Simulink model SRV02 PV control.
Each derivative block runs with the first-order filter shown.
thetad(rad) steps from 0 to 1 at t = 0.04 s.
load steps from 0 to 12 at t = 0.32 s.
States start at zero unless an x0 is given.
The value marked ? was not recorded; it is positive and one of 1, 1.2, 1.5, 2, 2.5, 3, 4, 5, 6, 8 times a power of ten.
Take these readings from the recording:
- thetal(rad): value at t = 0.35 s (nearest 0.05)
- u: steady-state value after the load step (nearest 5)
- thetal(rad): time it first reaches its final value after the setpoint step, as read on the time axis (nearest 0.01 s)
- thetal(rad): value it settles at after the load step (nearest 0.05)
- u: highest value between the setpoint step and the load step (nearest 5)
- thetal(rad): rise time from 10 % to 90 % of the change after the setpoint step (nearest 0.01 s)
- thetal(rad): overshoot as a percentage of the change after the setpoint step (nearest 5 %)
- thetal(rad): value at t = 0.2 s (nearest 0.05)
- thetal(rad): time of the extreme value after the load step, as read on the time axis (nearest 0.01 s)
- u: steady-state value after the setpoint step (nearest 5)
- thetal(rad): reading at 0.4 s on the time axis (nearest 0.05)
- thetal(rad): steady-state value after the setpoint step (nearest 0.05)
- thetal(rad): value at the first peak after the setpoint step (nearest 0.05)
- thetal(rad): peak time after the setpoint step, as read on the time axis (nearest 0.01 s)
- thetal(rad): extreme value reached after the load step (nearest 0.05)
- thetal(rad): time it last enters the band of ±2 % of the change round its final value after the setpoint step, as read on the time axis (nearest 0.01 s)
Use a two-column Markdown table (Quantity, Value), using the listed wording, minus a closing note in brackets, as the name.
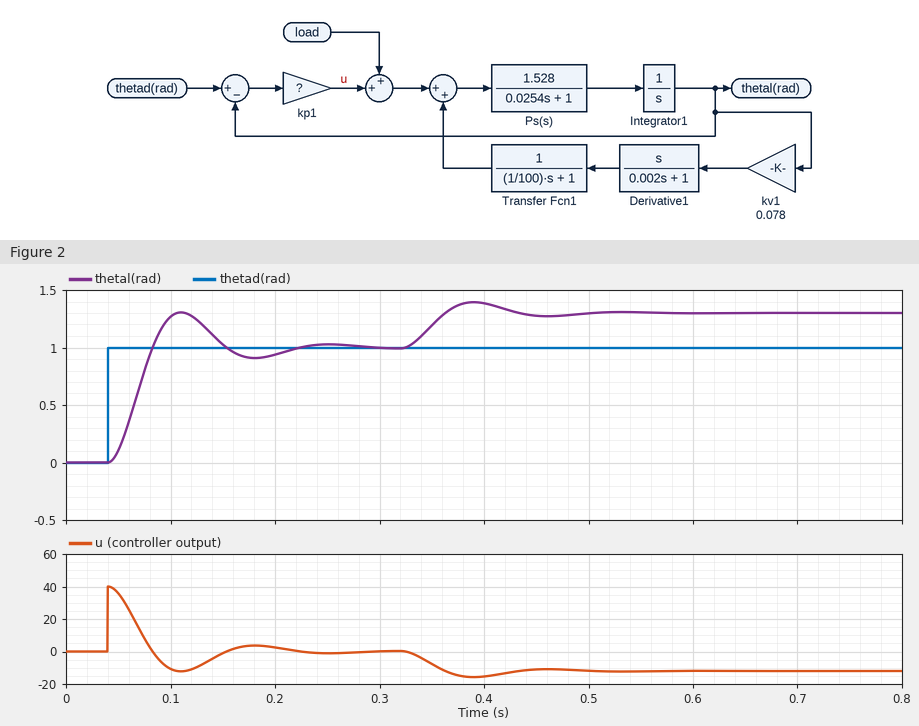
| Quantity | Value |
|---|---|
| thetal(rad): value at t = 0.35 s | 1.20 |
| u: steady-state value after the load step | -10 |
| thetal(rad): time it first reaches its final value after the setpoint step, as read on the time axis | 0.08 s |
| thetal(rad): value it settles at after the load step | 1.30 |
| u: highest value between the setpoint step and the load step | 40 |
| thetal(rad): rise time from 10 % to 90 % of the change after the setpoint step | 0.03 s |
| thetal(rad): overshoot as a percentage of the change after the setpoint step | 30 % |
| thetal(rad): value at t = 0.2 s | 0.95 |
| thetal(rad): time of the extreme value after the load step, as read on the time axis | 0.39 s |
| u: steady-state value after the setpoint step | 0 |
| thetal(rad): reading at 0.4 s on the time axis | 1.40 |
| thetal(rad): steady-state value after the setpoint step | 1.00 |
| thetal(rad): value at the first peak after the setpoint step | 1.30 |
| thetal(rad): peak time after the setpoint step, as read on the time axis | 0.11 s |
| thetal(rad): extreme value reached after the load step | 1.40 |
| thetal(rad): time it last enters the band of ±2 % of the change round its final value after the setpoint step, as read on the time axis | 0.27 s |
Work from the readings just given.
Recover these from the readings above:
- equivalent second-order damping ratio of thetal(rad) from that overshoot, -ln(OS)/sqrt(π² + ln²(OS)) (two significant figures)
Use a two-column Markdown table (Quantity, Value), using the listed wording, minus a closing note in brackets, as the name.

| Quantity | Value |
|---|---|
| equivalent second-order damping ratio of thetal(rad) from that overshoot, -ln(OS)/sqrt(π² + ln²(OS)) | 0.36 |
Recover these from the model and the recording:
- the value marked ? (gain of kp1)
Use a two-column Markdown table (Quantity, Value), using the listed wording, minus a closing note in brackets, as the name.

| Quantity | Value |
|---|---|
| the value marked ? | 40 |
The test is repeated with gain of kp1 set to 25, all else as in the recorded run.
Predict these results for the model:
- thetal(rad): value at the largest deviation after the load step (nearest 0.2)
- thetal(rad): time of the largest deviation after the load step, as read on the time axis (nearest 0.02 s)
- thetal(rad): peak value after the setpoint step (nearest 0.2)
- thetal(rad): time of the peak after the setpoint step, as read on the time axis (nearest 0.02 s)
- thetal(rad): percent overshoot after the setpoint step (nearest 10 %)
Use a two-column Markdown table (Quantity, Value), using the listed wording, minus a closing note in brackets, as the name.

| Quantity | Value |
|---|---|
| thetal(rad): value at the largest deviation after the load step | 1.6 |
| thetal(rad): time of the largest deviation after the load step, as read on the time axis | 0.42 s |
| thetal(rad): peak value after the setpoint step | 1.2 |
| thetal(rad): time of the peak after the setpoint step, as read on the time axis | 0.14 s |
| thetal(rad): percent overshoot after the setpoint step | 20 % |
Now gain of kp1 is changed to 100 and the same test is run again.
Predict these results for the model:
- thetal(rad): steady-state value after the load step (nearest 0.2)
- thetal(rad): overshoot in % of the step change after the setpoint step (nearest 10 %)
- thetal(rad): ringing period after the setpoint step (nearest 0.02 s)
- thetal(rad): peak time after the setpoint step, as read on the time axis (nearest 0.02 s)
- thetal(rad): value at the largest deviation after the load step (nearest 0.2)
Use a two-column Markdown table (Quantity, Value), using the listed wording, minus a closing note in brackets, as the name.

| Quantity | Value |
|---|---|
| thetal(rad): steady-state value after the load step | 1.2 |
| thetal(rad): overshoot in % of the step change after the setpoint step | 50 % |
| thetal(rad): ringing period after the setpoint step | 0.08 s |
| thetal(rad): peak time after the setpoint step, as read on the time axis | 0.08 s |
| thetal(rad): value at the largest deviation after the load step | 1.2 |
